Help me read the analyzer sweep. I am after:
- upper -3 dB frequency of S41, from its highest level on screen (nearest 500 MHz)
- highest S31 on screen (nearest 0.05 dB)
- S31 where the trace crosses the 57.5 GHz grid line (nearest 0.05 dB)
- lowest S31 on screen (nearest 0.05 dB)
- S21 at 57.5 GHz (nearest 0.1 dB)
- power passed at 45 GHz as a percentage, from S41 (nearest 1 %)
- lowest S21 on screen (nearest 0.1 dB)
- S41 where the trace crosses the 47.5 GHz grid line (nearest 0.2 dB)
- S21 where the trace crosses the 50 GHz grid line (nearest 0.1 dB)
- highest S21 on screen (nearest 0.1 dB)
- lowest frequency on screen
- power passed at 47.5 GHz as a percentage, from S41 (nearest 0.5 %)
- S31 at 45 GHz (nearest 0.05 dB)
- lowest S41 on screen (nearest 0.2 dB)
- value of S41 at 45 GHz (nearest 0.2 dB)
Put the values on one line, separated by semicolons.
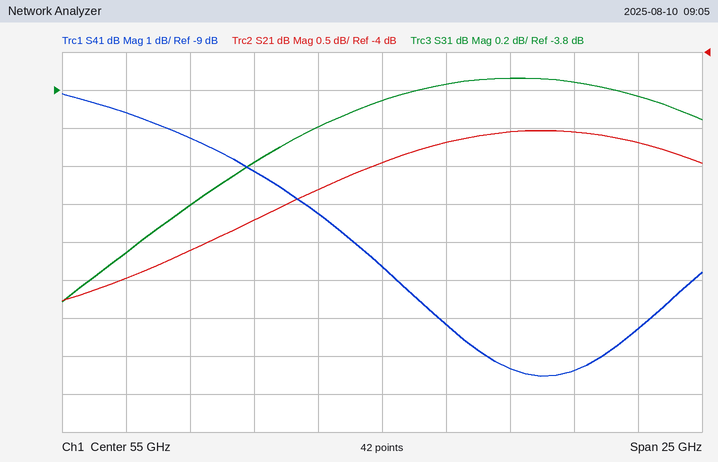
52.0 GHz; -3.75 dB; -3.75 dB; -4.90 dB; -5.2 dB; 11 %; -7.3 dB; -10.2 dB; -6.2 dB; -5.0 dB; 42.5 GHz; 9.5 %; -4.65 dB; -16.6 dB; -9.6 dB
